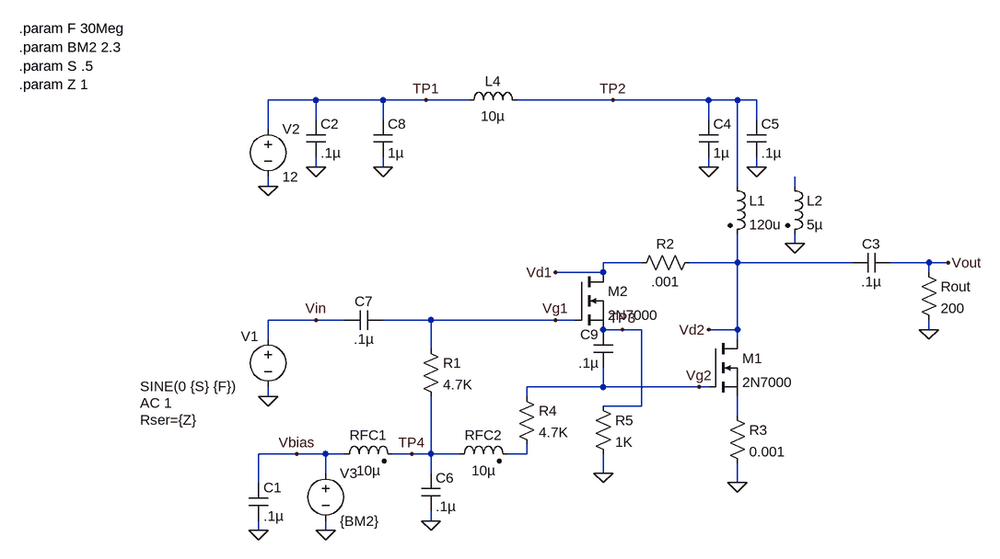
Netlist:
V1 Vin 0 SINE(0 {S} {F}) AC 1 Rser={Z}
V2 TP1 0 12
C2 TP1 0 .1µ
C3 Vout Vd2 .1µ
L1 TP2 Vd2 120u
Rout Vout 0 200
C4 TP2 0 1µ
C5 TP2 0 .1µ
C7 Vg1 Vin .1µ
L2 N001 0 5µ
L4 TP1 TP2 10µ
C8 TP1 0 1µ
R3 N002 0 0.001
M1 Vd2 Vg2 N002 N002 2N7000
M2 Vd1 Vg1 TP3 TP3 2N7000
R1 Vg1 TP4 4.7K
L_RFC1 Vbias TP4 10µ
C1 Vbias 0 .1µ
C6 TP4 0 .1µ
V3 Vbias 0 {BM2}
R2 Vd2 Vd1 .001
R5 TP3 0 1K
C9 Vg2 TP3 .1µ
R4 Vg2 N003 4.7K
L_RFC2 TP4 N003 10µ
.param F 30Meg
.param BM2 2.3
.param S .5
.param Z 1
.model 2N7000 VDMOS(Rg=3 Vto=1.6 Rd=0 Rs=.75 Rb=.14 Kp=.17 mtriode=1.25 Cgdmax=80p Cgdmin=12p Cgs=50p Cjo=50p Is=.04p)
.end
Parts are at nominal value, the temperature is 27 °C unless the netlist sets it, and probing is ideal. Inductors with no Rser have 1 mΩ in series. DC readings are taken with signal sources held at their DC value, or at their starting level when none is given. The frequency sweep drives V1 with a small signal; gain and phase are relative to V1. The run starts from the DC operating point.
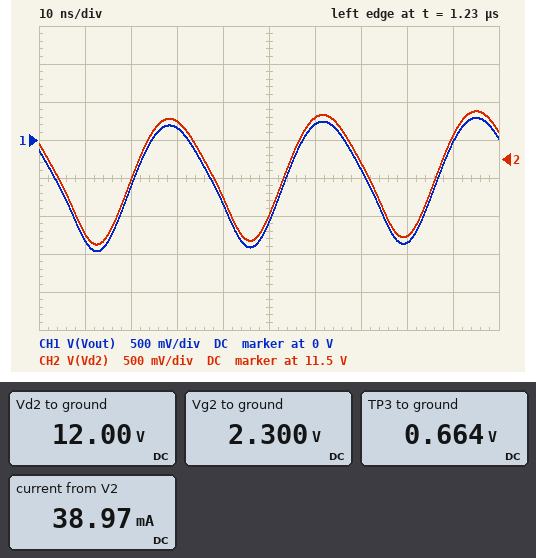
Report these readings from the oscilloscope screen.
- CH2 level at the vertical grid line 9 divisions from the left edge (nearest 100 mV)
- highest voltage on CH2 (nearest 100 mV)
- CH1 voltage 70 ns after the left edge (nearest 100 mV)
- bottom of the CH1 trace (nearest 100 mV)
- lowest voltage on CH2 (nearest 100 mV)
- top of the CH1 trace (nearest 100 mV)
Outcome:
11.8 V
12.1 V
-400 mV
-1.5 V
10.4 V
300 mV
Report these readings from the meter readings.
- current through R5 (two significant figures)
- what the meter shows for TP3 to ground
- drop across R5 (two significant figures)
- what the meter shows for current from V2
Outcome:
660 µA
0.664 V
660 mV
38.97 mA
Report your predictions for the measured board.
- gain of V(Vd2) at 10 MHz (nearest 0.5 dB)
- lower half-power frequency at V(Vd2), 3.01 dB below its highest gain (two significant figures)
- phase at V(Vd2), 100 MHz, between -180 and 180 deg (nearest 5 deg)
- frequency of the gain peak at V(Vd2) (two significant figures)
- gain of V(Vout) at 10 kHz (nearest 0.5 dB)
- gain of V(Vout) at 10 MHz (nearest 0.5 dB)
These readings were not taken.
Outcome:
12.0 dB
47 kHz
95 deg
48 kHz
-4.5 dB
12.0 dB
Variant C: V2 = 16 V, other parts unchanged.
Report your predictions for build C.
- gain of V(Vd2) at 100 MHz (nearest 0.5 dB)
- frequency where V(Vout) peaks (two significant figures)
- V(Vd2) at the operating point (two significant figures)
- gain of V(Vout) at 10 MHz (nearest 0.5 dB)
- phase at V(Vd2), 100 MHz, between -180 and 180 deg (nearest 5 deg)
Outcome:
2.0 dB
760 kHz
16 V
13.0 dB
95 deg
